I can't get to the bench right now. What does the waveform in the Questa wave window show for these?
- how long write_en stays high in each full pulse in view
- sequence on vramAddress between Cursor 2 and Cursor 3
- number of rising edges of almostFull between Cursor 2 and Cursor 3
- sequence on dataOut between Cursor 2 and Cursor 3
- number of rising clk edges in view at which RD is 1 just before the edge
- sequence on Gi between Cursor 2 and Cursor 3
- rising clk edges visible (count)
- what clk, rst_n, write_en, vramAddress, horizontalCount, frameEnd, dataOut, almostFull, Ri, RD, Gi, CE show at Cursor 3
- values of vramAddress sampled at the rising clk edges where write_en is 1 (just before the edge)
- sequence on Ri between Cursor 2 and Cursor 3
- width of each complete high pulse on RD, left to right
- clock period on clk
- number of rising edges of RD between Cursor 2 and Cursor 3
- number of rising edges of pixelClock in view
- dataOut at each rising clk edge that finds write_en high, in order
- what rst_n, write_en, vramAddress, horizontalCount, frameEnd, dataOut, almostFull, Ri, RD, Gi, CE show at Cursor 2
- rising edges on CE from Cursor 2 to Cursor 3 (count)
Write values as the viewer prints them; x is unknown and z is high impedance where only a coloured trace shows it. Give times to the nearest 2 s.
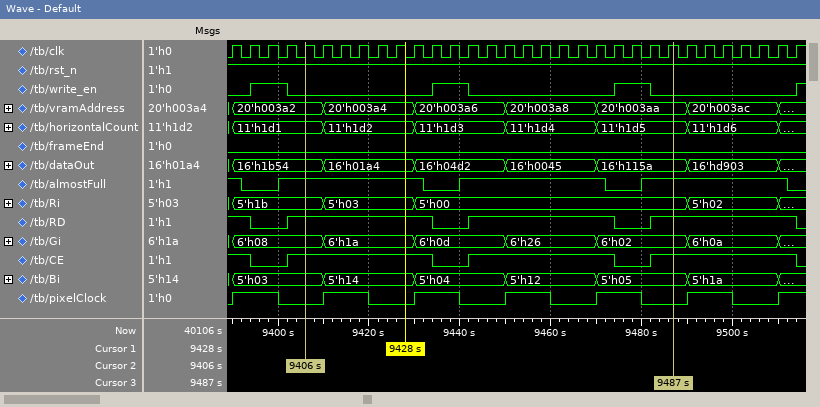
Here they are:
8 s, 8 s, 8 s
20'h003a2, 20'h003a4, 20'h003a6, 20'h003a8, 20'h003aa
2
16'h1b54, 16'h01a4, 16'h04d2, 16'h0045, 16'h115a
26
6'h08, 6'h1a, 6'h0d, 6'h26, 6'h02
32
clk=1, rst_n=1, write_en=0, vramAddress=20'h003aa, horizontalCount=11'h1d5, frameEnd=0, dataOut=16'h115a, almostFull=1, Ri=5'h00, RD=1, Gi=6'h02, CE=1
20'h003a2, 20'h003a2, 20'h003a6, 20'h003a6, 20'h003aa, 20'h003aa
5'h1b, 5'h03, 5'h00
32 s, 32 s, 32 s
4 s
2
7
16'h1b54, 16'h1b54, 16'h04d2, 16'h04d2, 16'h115a, 16'h115a
rst_n=1, write_en=0, vramAddress=20'h003a2, horizontalCount=11'h1d1, frameEnd=0, dataOut=16'h1b54, almostFull=1, Ri=5'h1b, RD=1, Gi=6'h08, CE=1
2
